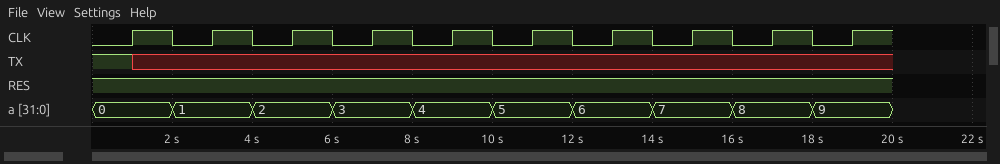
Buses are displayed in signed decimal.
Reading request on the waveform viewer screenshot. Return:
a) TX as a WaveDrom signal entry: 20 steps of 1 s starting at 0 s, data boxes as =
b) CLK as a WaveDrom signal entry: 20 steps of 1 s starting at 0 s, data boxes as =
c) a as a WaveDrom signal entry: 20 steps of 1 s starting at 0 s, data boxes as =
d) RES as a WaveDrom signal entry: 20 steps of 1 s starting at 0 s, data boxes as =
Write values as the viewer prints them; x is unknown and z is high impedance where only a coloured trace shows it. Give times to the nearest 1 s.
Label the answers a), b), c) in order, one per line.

a) {name: 'TX', wave: '1x..................'}
b) {name: 'CLK', wave: '01010101010101010101'}
c) {name: 'a', wave: '=.=.=.=.=.=.=.=.=.=.', data: '0 1 2 3 4 5 6 7 8 9'}
d) {name: 'RES', wave: '1...................'}
